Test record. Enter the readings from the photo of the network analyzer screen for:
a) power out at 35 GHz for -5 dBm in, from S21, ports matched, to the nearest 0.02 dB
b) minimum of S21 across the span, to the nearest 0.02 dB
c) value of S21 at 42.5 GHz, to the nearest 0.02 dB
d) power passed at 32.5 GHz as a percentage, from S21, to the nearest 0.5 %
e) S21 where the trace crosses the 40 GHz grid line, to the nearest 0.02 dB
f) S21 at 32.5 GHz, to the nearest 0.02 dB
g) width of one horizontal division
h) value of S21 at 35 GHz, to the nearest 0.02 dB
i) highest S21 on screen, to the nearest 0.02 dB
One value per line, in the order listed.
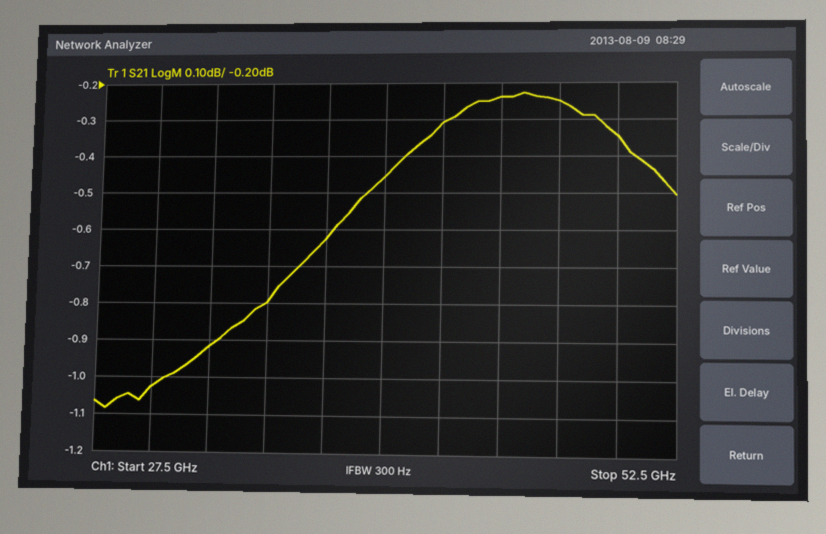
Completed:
-5.80 dBm
-1.08 dB
-0.30 dB
81.0 %
-0.46 dB
-0.92 dB
2.5 GHz
-0.80 dB
-0.22 dB
